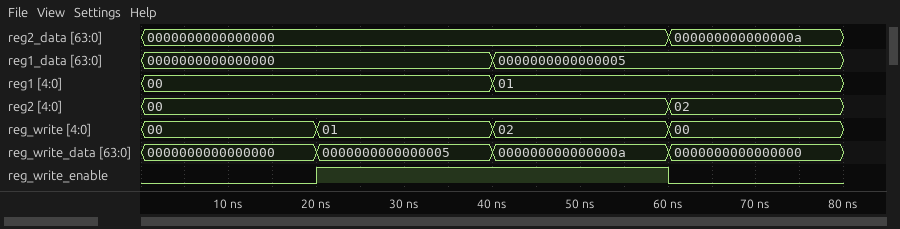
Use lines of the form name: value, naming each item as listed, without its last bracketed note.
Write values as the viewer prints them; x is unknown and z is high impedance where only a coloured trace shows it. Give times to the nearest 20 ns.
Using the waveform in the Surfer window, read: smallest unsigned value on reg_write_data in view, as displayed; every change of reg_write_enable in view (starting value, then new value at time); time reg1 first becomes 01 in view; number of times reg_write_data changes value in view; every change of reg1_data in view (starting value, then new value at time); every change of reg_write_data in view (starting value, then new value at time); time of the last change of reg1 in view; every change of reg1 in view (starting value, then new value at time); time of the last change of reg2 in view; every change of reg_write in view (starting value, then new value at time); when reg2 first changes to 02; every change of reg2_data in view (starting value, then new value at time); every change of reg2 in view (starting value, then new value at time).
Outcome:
smallest unsigned value on reg_write_data in view, as displayed: 0000000000000000
every change of reg_write_enable in view: 0, 1 at 20 ns, 0 at 60 ns
time reg1 first becomes 01 in view: 40 ns
number of times reg_write_data changes value in view: 3
every change of reg1_data in view: 0000000000000000, 0000000000000005 at 40 ns
every change of reg_write_data in view: 0000000000000000, 0000000000000005 at 20 ns, 000000000000000a at 40 ns, 0000000000000000 at 60 ns
time of the last change of reg1 in view: 40 ns
every change of reg1 in view: 00, 01 at 40 ns
time of the last change of reg2 in view: 60 ns
every change of reg_write in view: 00, 01 at 20 ns, 02 at 40 ns, 00 at 60 ns
when reg2 first changes to 02: 60 ns
every change of reg2_data in view: 0000000000000000, 000000000000000a at 60 ns
every change of reg2 in view: 00, 02 at 60 ns
